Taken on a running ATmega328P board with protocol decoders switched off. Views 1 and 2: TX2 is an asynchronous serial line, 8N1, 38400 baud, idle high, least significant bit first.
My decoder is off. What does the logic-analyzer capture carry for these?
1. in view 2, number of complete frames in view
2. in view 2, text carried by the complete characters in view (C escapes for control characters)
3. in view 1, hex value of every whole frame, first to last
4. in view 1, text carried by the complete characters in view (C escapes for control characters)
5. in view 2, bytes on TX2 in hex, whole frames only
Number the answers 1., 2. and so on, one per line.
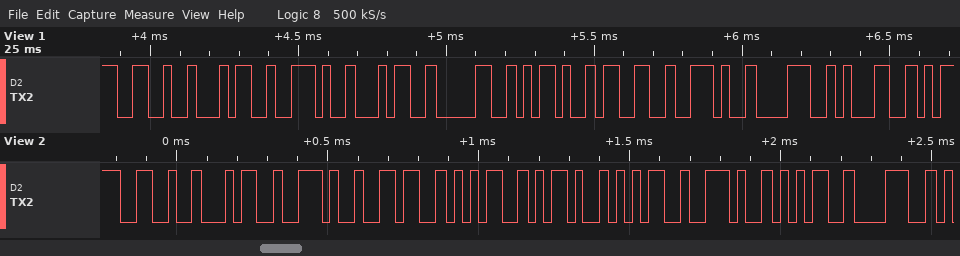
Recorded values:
1. 10
2. "&4.65-5.58"
3. 26 34 2E 34 30 2D 33 2E 38 31
4. "&4.40-3.81"
5. 26 34 2E 36 35 2D 35 2E 35 38
